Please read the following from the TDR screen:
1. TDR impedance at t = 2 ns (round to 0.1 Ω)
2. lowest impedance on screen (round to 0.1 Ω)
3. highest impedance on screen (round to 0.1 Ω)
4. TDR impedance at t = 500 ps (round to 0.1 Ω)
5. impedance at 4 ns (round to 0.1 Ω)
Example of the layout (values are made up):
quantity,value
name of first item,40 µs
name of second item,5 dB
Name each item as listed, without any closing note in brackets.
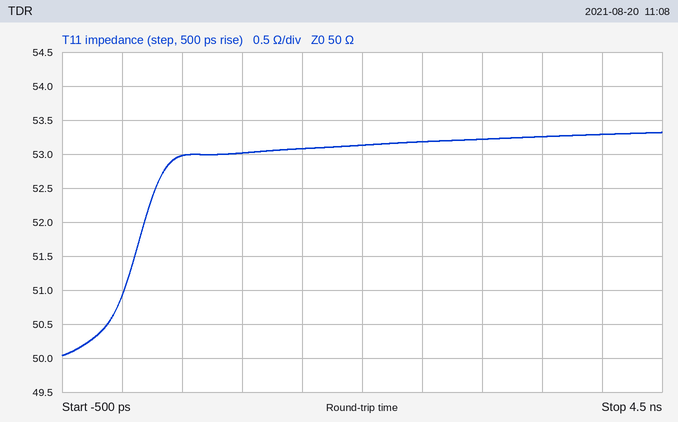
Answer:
quantity,value
TDR impedance at t = 2 ns,53.1 Ω
lowest impedance on screen,50.0 Ω
highest impedance on screen,53.3 Ω
TDR impedance at t = 500 ps,53.0 Ω
impedance at 4 ns,53.3 Ω
